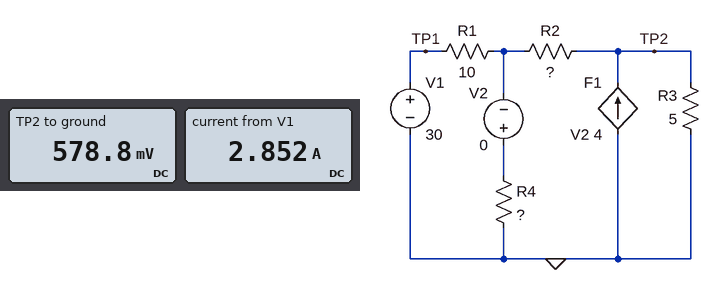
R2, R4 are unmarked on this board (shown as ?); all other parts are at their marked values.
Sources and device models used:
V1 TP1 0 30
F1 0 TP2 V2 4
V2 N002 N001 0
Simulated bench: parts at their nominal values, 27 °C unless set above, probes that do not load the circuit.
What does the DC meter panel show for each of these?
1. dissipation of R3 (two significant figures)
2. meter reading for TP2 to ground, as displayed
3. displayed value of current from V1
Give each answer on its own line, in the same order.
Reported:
67 mW
578.8 mV
2.852 A
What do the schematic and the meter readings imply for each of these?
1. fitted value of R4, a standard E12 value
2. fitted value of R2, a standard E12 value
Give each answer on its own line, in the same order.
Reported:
2.7 Ω
0.39 Ω
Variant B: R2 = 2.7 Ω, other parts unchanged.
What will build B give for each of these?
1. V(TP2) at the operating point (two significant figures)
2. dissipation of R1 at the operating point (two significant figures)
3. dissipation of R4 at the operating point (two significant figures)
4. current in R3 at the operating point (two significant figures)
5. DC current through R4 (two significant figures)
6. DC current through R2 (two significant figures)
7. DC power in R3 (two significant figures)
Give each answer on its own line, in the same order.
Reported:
-3.7 V
79 W
1.4 W
750 mA
710 mA
2.1 A
2.8 W
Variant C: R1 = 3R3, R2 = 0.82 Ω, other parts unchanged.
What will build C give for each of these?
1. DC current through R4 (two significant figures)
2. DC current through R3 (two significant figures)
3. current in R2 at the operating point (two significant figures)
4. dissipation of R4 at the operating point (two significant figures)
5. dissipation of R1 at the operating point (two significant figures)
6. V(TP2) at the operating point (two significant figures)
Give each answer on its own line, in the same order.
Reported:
1.6 A
160 mA
6.2 A
6.8 W
200 W
-790 mV
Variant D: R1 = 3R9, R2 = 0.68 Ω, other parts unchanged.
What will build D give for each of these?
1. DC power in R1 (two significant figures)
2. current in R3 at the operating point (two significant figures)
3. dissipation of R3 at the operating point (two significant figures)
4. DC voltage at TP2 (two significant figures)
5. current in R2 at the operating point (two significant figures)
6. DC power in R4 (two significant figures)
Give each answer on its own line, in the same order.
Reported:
180 W
4.8 mA
110 µW
-24 mV
5.4 A
4.9 W
